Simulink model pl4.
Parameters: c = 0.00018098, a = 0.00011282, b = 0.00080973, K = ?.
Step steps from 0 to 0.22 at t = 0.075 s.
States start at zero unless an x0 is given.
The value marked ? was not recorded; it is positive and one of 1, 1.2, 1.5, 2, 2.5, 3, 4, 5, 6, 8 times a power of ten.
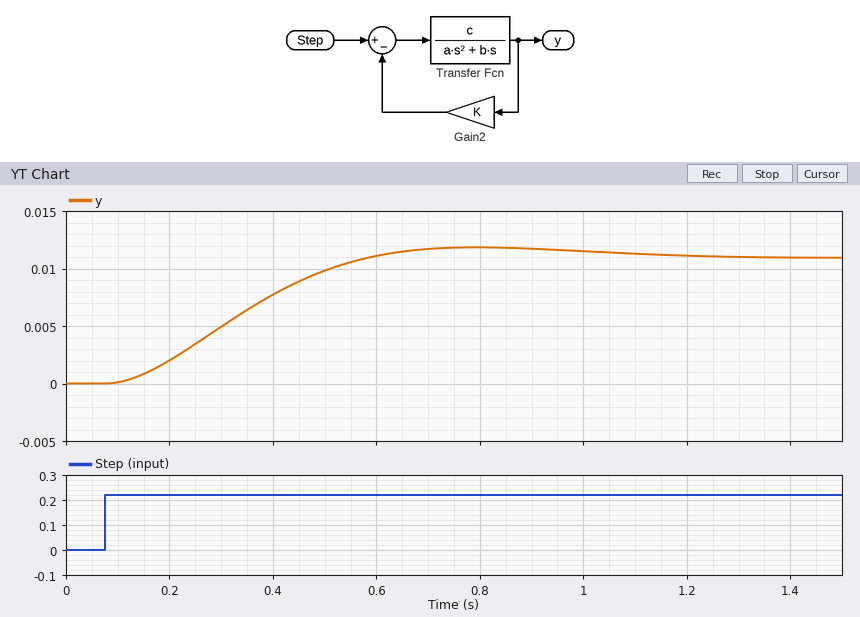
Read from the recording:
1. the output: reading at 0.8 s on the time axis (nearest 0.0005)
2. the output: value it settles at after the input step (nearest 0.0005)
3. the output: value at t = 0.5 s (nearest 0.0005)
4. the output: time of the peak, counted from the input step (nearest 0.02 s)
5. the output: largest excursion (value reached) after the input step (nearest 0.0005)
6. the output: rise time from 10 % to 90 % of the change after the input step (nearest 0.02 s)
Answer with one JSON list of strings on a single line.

["0.0120", "0.0110", "0.0100", "0.72 s", "0.0120", "0.34 s"]
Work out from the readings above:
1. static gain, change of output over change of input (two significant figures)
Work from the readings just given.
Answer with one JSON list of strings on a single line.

["0.050"]
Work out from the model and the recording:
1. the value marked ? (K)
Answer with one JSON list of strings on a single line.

["20"]
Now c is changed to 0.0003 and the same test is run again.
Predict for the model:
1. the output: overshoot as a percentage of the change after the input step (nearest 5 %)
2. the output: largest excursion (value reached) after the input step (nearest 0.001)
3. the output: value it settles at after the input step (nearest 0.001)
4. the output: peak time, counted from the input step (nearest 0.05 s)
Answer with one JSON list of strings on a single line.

["15 %", "0.013", "0.011", "0.50 s"]
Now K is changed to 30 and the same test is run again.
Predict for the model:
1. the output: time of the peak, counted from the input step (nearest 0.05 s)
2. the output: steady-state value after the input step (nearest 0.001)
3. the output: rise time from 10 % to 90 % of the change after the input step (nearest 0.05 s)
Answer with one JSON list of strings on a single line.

["0.55 s", "0.007", "0.25 s"]
